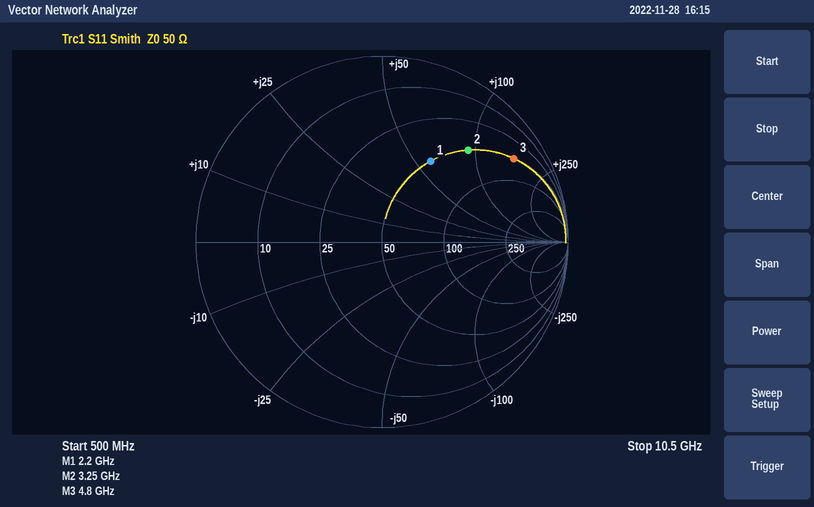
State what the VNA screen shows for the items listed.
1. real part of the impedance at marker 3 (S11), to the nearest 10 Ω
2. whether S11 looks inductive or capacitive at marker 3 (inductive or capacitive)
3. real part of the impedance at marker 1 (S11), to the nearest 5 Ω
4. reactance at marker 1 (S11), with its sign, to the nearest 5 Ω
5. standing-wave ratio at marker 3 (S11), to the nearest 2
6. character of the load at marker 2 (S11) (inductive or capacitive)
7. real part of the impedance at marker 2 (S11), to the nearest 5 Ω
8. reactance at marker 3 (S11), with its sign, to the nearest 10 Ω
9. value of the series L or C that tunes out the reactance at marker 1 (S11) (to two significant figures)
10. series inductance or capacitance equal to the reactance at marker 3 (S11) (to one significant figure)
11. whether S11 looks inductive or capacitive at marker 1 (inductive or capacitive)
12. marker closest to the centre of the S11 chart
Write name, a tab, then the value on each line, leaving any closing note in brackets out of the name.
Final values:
real part of the impedance at marker 3 (S11), to the nearest 10 Ω	50 Ω
whether S11 looks inductive or capacitive at marker 3	inductive
real part of the impedance at marker 1 (S11), to the nearest 5 Ω	50 Ω
reactance at marker 1 (S11), with its sign, to the nearest 5 Ω	+60 Ω
standing-wave ratio at marker 3 (S11), to the nearest 2	12
character of the load at marker 2 (S11)	inductive
real part of the impedance at marker 2 (S11), to the nearest 5 Ω	50 Ω
reactance at marker 3 (S11), with its sign, to the nearest 10 Ω	+160 Ω
value of the series L or C that tunes out the reactance at marker 1 (S11)	1.2 pF
series inductance or capacitance equal to the reactance at marker 3 (S11)	5 nH
whether S11 looks inductive or capacitive at marker 1	inductive
marker closest to the centre of the S11 chart	marker 1
